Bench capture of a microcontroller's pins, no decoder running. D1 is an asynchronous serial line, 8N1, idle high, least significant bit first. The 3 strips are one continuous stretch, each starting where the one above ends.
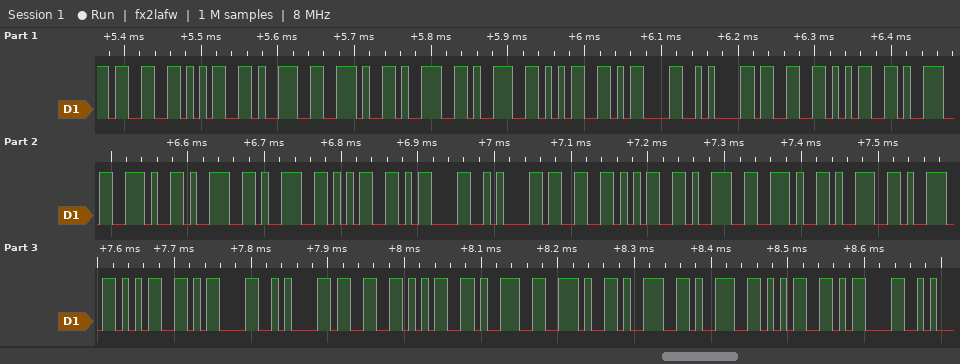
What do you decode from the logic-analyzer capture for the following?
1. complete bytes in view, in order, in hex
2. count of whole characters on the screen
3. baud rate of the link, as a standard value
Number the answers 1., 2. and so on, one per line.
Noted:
1. 33 35 39 2E 39 39 35 0D 0A 33 35 39 2E 39 39 35 0D 0A 33 35 39 2E 39 39 35 0D 0A 33 35 39 2E 39 39 35 0D
2. 35
3. 115200 baud
